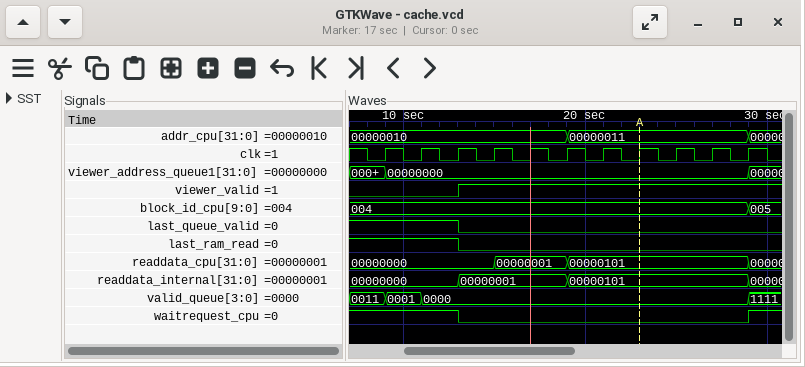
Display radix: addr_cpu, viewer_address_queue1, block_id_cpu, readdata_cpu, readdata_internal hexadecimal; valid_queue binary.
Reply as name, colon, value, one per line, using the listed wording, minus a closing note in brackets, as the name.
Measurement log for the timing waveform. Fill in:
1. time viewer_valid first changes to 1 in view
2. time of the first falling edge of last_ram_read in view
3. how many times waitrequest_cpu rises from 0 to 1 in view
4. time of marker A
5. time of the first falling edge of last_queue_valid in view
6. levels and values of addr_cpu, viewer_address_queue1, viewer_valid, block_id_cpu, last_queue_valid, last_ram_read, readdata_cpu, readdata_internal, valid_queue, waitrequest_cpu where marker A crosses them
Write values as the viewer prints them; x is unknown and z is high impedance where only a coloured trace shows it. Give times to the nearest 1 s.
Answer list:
time viewer_valid first changes to 1 in view: 13 s
time of the first falling edge of last_ram_read in view: 13 s
how many times waitrequest_cpu rises from 0 to 1 in view: 1
time of marker A: 23 s
time of the first falling edge of last_queue_valid in view: 13 s
levels and values of addr_cpu, viewer_address_queue1, viewer_valid, block_id_cpu, last_queue_valid, last_ram_read, readdata_cpu, readdata_internal, valid_queue, waitrequest_cpu where marker A crosses them: addr_cpu=00000011, viewer_address_queue1=00000000, viewer_valid=1, block_id_cpu=004, last_queue_valid=0, last_ram_read=0, readdata_cpu=00000101, readdata_internal=00000101, valid_queue=0000, waitrequest_cpu=0
